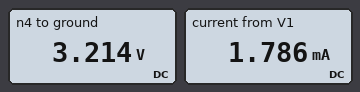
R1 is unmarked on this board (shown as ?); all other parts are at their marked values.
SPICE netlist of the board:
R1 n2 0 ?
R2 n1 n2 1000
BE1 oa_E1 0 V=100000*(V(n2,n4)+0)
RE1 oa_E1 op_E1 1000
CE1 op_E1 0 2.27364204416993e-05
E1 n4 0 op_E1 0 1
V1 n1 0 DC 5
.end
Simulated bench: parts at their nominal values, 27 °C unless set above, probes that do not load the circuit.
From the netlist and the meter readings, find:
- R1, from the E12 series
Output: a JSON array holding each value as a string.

["1.8 kΩ"]
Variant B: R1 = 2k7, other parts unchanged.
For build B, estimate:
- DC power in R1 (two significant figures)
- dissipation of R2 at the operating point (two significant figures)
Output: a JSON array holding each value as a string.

["4.9 mW", "1.8 mW"]
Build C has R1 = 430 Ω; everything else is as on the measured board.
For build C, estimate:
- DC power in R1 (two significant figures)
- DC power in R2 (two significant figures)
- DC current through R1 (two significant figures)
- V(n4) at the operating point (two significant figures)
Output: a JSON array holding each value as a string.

["5.3 mW", "12 mW", "3.5 mA", "1.5 V"]
